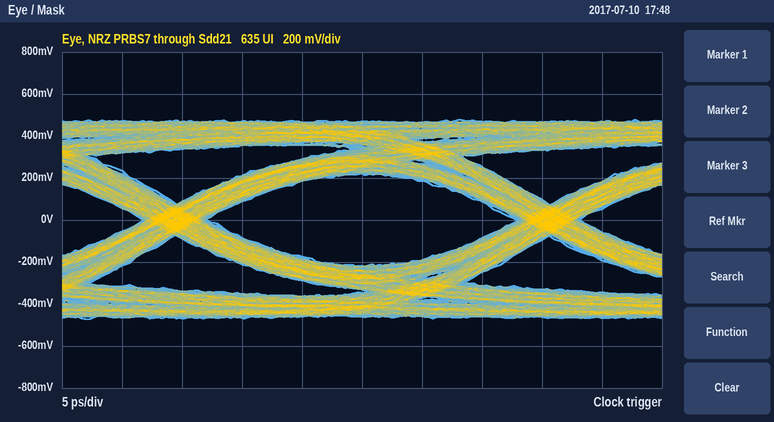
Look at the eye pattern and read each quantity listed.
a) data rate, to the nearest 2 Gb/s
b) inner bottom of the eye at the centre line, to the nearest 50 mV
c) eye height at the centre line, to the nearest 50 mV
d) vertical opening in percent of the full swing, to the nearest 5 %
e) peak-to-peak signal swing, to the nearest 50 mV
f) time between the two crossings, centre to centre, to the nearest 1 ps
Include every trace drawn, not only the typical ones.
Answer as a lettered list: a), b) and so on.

a) 32 Gb/s
b) -200 mV
c) 450 mV
d) 45 %
e) 950 mV
f) 31 ps
